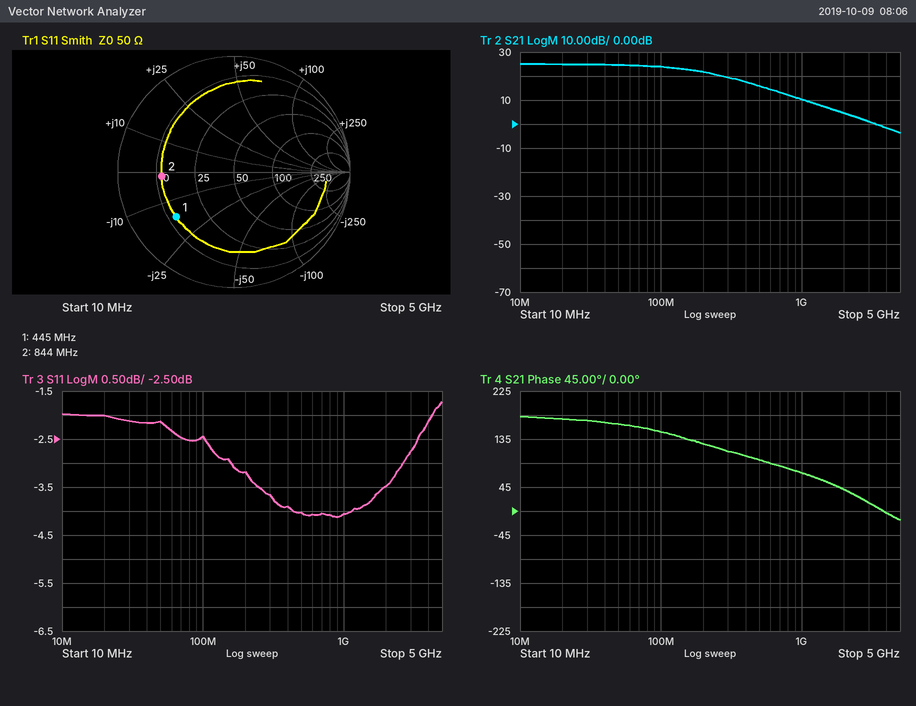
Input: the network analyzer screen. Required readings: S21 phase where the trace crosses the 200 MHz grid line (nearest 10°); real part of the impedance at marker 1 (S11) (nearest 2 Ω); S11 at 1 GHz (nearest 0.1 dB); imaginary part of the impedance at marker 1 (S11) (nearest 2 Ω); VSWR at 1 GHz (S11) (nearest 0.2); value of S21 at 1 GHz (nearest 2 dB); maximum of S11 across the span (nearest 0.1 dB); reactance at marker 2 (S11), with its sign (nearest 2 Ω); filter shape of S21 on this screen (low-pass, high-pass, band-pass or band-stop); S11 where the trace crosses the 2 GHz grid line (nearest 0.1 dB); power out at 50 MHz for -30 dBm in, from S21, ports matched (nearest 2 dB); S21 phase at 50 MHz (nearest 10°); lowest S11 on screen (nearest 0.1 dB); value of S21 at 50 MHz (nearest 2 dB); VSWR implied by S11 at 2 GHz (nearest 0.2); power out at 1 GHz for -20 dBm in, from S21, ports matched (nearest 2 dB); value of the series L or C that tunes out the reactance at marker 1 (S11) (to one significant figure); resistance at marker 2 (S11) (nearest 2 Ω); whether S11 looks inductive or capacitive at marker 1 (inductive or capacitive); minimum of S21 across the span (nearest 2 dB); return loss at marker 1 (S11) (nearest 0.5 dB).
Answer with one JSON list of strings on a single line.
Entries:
["130°", "12 Ω", "-4.1 dB", "-16 Ω", "4.4", "10 dB", "-1.7 dB", "-2 Ω", "low-pass", "-3.5 dB", "-6 dBm", "160°", "-4.1 dB", "24 dB", "5.0", "-10 dBm", "6 nH", "12 Ω", "capacitive", "-4 dB", "4.0 dB"]
